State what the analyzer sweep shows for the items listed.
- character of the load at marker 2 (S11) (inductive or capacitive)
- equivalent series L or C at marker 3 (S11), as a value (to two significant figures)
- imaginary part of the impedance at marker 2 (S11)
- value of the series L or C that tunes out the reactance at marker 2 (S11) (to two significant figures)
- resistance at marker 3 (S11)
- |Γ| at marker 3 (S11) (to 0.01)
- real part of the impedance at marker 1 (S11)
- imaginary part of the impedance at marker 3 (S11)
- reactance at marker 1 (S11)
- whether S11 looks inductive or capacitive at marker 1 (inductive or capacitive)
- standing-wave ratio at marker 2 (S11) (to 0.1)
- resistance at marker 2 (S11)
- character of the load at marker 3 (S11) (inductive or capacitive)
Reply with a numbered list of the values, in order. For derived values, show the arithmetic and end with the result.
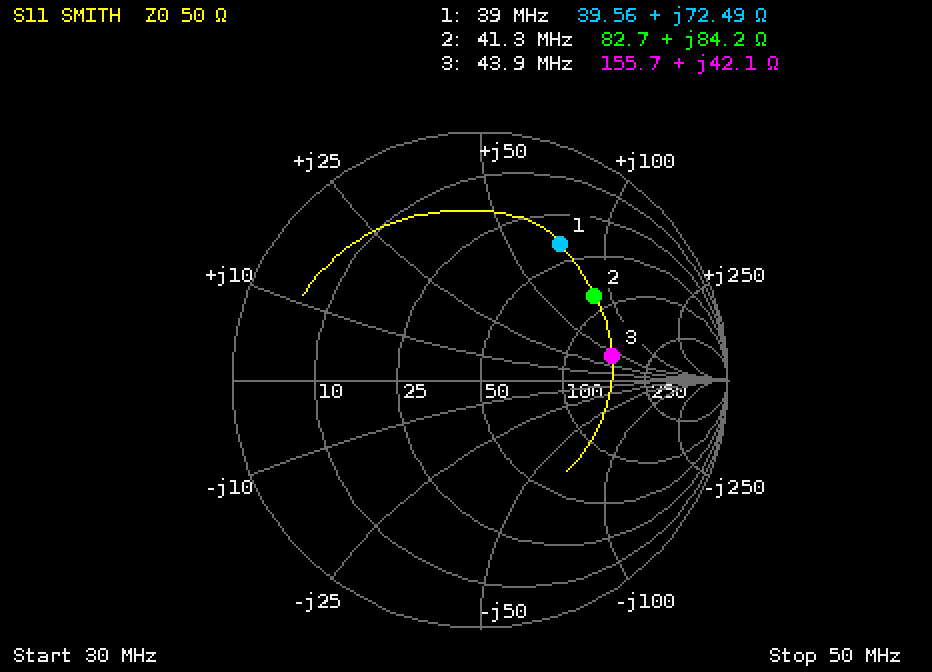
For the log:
1. inductive
2. L = 42.1 Ω/(2π × 43.9 MHz) ≈ 153 nH, so 150 nH to two significant figures
3. +84.2 Ω
4. C = 1/(2π × 41.3 MHz × 84.2 Ω) ≈ 46 pF
5. 155.7 Ω
6. 0.54
7. 39.56 Ω
8. +42.1 Ω
9. +72.49 Ω
10. inductive
11. 3.7
12. 82.7 Ω
13. inductive
